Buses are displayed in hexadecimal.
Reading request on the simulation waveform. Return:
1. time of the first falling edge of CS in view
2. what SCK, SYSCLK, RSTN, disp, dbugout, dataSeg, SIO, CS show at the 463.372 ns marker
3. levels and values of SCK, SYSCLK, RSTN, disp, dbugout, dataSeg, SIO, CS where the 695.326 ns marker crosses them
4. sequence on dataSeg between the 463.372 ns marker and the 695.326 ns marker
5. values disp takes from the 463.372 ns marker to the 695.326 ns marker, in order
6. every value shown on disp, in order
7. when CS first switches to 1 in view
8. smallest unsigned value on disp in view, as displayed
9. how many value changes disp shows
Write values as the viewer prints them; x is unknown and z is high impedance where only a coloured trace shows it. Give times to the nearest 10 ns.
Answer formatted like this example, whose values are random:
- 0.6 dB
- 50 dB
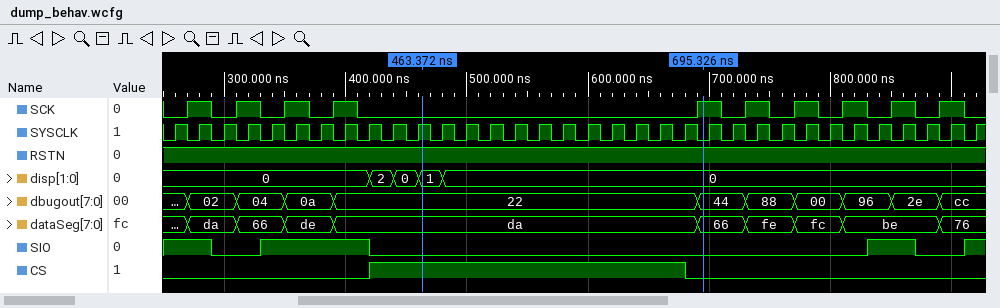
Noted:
- 680 ns
- SCK=0, SYSCLK=1, RSTN=1, disp=1, dbugout=22, dataSeg=da, SIO=0, CS=1
- SCK=1, SYSCLK=0, RSTN=1, disp=0, dbugout=44, dataSeg=66, SIO=0, CS=0
- da, 66
- 1, 0
- 0, 2, 0, 1, 0
- 420 ns
- 0
- 4
